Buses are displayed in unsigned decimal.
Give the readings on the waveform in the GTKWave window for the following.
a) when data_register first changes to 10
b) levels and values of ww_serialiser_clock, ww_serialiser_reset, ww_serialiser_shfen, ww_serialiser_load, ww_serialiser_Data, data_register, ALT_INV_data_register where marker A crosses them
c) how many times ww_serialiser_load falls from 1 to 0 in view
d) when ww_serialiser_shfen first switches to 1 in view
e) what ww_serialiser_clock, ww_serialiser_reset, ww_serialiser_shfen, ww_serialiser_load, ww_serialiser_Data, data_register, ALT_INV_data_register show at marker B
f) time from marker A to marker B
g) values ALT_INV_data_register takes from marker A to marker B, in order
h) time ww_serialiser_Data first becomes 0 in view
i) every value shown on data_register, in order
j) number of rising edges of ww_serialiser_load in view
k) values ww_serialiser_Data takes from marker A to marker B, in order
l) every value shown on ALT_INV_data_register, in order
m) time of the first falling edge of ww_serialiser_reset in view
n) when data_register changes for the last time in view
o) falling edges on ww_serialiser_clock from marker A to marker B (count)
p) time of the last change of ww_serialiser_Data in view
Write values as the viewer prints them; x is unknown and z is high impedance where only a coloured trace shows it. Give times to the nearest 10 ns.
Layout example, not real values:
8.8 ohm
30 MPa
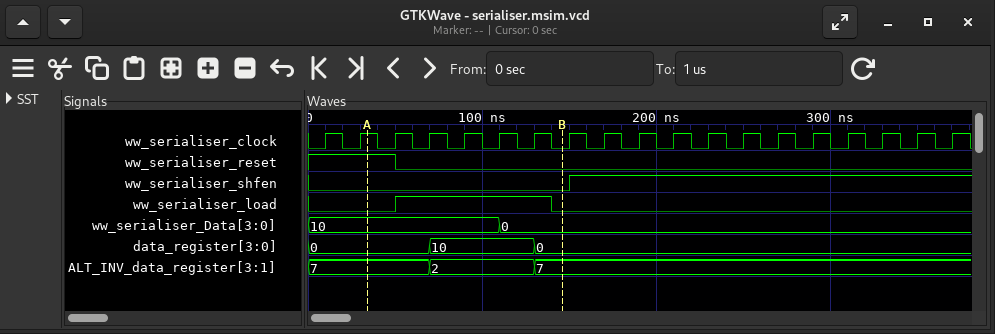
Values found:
70 ns
ww_serialiser_clock=1, ww_serialiser_reset=1, ww_serialiser_shfen=0, ww_serialiser_load=0, ww_serialiser_Data=10, data_register=0, ALT_INV_data_register=7
1
150 ns
ww_serialiser_clock=0, ww_serialiser_reset=0, ww_serialiser_shfen=0, ww_serialiser_load=0, ww_serialiser_Data=0, data_register=0, ALT_INV_data_register=7
110 ns
7, 2, 7
110 ns
0, 10, 0
1
10, 0
7, 2, 7
50 ns
130 ns
6
110 ns
